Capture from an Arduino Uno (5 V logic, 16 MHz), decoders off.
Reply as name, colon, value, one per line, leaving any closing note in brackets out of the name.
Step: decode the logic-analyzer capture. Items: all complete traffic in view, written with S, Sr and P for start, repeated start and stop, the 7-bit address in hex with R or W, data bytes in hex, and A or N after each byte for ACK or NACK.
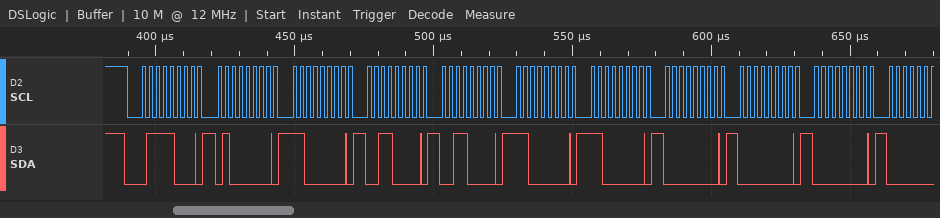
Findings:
all complete traffic in view, written with S, Sr and P for start, repeated start and stop, the 7-bit address in hex with R or W, data bytes in hex, and A or N after each byte for ACK or NACK: S 3CW A 40 A C0 A 30 A 30 A C0 A C0 A 00 A 00 A 00 A
